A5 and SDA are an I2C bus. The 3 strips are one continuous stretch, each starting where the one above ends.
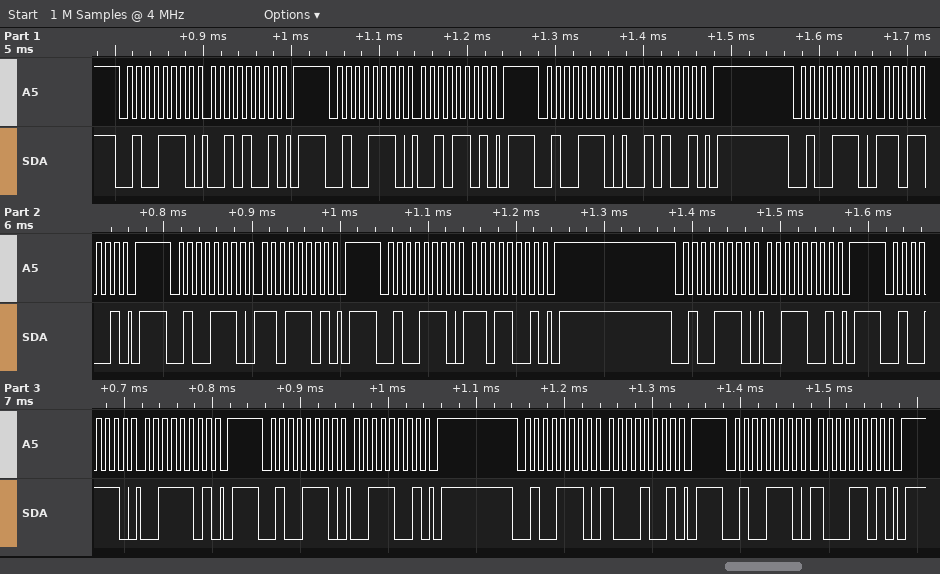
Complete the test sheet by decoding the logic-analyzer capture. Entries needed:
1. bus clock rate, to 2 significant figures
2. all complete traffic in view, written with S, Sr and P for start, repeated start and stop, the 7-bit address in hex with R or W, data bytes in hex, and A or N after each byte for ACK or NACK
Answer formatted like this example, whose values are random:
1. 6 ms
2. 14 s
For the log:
1. 100 kHz
2. S 27W A 29 A P S 27W A 2D A P S 27W A 29 A P S 27W A D9 A P S 27W A DD A P S 27W A D9 A P S 27W A 39 A P S 27W A 3D A P S 27W A 39 A P S 27W A 89 A P S 27W A 8D A P
